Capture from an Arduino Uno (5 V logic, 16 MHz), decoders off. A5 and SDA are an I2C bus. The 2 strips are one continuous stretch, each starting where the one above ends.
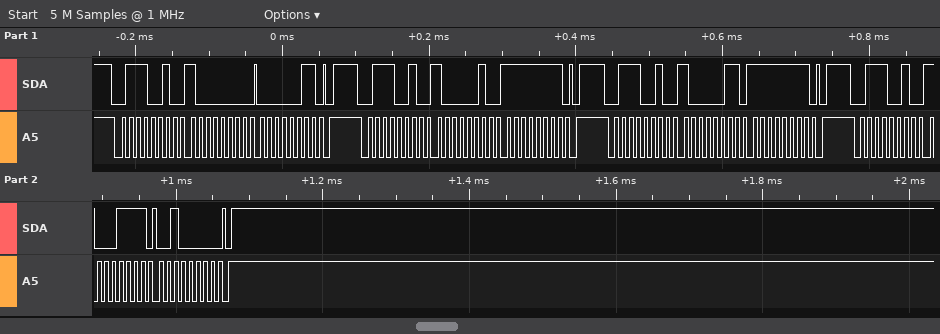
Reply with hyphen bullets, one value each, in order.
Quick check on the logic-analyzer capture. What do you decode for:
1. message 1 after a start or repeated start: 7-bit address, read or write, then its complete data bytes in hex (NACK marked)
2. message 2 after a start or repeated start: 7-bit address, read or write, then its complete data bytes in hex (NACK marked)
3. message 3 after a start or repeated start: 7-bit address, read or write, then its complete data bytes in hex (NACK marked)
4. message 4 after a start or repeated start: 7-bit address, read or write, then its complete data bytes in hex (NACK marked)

- 0x39 write: 80 03
- 0x39 write: 82 FF
- 0x39 write: 83 FF
- 0x39 write: 8F 20
